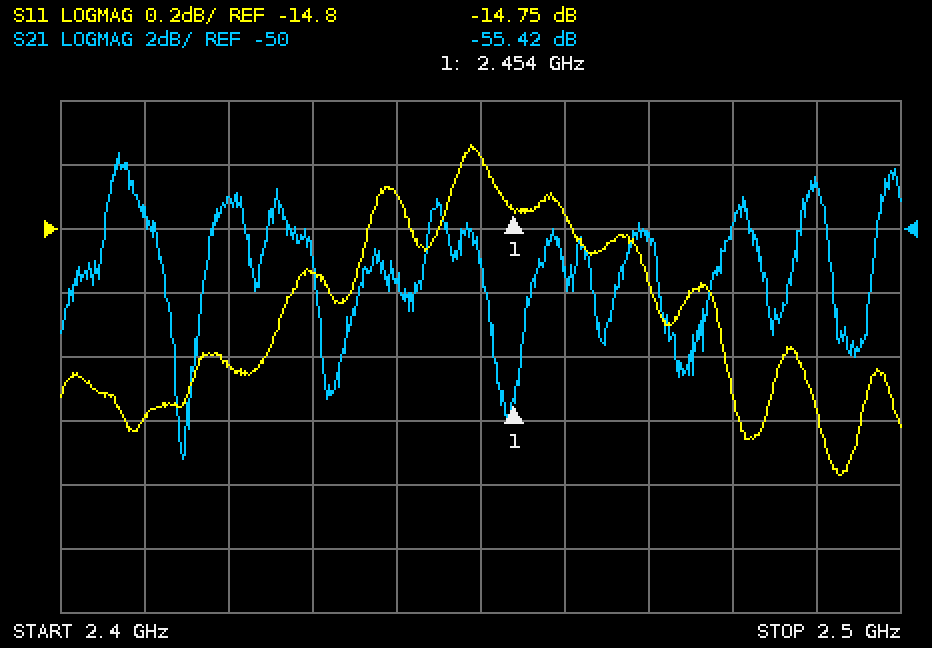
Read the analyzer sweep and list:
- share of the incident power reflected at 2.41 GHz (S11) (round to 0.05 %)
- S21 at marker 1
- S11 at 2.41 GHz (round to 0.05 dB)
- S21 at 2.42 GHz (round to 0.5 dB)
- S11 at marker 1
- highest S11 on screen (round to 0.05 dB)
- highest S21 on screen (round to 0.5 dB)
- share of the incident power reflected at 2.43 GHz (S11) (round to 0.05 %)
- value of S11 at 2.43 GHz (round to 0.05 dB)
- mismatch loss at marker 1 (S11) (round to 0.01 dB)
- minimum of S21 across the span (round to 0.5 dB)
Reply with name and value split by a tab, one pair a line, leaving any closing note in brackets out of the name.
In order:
share of the incident power reflected at 2.41 GHz (S11)	2.90 %
S21 at marker 1	-55.42 dB
S11 at 2.41 GHz	-15.40 dB
S21 at 2.42 GHz	-49.0 dB
S11 at marker 1	-14.75 dB
highest S11 on screen	-14.55 dB
highest S21 on screen	-47.5 dB
share of the incident power reflected at 2.43 GHz (S11)	3.20 %
value of S11 at 2.43 GHz	-14.95 dB
mismatch loss at marker 1 (S11)	0.15 dB
minimum of S21 across the span	-57.0 dB
